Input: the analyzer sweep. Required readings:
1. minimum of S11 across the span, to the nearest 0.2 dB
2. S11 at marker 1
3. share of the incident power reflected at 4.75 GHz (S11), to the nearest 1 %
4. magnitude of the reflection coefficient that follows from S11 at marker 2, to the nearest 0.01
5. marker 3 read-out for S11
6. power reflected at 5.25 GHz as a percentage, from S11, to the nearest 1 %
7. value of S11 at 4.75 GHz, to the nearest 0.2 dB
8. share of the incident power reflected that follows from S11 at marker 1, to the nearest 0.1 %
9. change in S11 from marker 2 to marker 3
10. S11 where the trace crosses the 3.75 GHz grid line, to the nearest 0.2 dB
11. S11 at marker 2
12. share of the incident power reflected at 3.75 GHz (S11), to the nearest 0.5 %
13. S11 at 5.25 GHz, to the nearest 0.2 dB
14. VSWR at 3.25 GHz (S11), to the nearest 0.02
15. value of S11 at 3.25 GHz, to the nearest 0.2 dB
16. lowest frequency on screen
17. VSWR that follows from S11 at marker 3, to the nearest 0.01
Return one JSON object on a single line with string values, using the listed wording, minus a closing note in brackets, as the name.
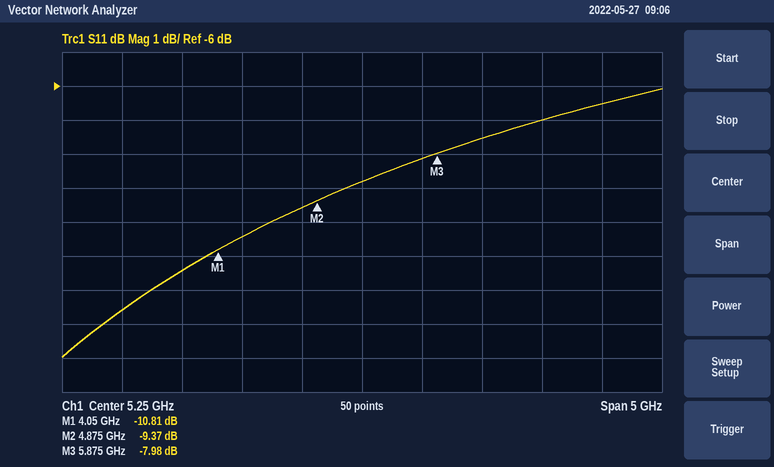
{"minimum of S11 across the span, to the nearest 0.2 dB": "-14.0 dB", "S11 at marker 1": "-10.81 dB", "share of the incident power reflected at 4.75 GHz (S11), to the nearest 1 %": "11 %", "magnitude of the reflection coefficient that follows from S11 at marker 2, to the nearest 0.01": "0.34", "marker 3 read-out for S11": "-7.98 dB", "power reflected at 5.25 GHz as a percentage, from S11, to the nearest 1 %": "13 %", "value of S11 at 4.75 GHz, to the nearest 0.2 dB": "-9.6 dB", "share of the incident power reflected that follows from S11 at marker 1, to the nearest 0.1 %": "8.3 %", "change in S11 from marker 2 to marker 3": "1.39 dB", "S11 where the trace crosses the 3.75 GHz grid line, to the nearest 0.2 dB": "-11.4 dB", "S11 at marker 2": "-9.37 dB", "share of the incident power reflected at 3.75 GHz (S11), to the nearest 0.5 %": "7.0 %", "S11 at 5.25 GHz, to the nearest 0.2 dB": "-8.8 dB", "VSWR at 3.25 GHz (S11), to the nearest 0.02": "1.62", "value of S11 at 3.25 GHz, to the nearest 0.2 dB": "-12.6 dB", "lowest frequency on screen": "2.75 GHz", "VSWR that follows from S11 at marker 3, to the nearest 0.01": "2.33"}
